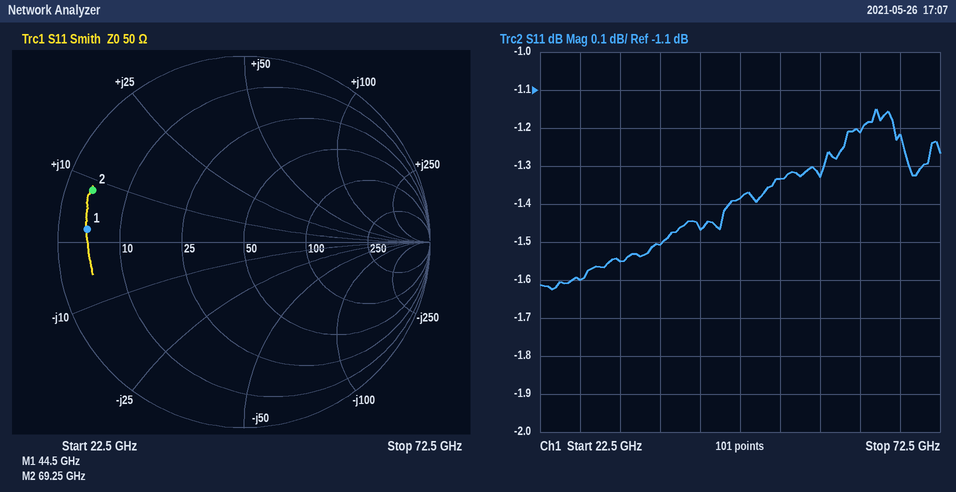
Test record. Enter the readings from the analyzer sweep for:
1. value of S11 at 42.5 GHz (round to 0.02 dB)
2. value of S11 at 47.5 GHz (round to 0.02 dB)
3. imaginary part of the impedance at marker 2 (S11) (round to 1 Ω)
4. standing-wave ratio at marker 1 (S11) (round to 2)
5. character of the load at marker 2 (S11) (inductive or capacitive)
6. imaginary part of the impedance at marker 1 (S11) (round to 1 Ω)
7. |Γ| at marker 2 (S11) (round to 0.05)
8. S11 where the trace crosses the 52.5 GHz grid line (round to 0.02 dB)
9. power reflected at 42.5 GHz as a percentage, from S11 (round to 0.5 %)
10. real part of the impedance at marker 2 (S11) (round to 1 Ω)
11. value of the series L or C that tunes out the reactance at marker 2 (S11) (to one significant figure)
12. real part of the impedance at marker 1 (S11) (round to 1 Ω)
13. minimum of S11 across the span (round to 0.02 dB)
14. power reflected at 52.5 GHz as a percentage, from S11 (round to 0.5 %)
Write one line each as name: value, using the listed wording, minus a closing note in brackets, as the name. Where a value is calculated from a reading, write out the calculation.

value of S11 at 42.5 GHz: -1.46 dB
value of S11 at 47.5 GHz: -1.38 dB
imaginary part of the impedance at marker 2 (S11): +8 Ω
standing-wave ratio at marker 1 (S11): 12
character of the load at marker 2 (S11): inductive
imaginary part of the impedance at marker 1 (S11): +2 Ω
|Γ| at marker 2 (S11): 0.85
S11 where the trace crosses the 52.5 GHz grid line: -1.34 dB
power reflected at 42.5 GHz as a percentage, from S11: 10^(-1.46/10) ≈ 71.4 %, so 71.5 % to the nearest 0.5 %
real part of the impedance at marker 2 (S11): 4 Ω
value of the series L or C that tunes out the reactance at marker 2 (S11): C = 1/(2π × 69.25 GHz × 8 Ω) ≈ 287 fF, so 300 fF to one significant figure
real part of the impedance at marker 1 (S11): 4 Ω
minimum of S11 across the span: -1.62 dB
power reflected at 52.5 GHz as a percentage, from S11: 10^(-1.34/10) ≈ 73.5 %
